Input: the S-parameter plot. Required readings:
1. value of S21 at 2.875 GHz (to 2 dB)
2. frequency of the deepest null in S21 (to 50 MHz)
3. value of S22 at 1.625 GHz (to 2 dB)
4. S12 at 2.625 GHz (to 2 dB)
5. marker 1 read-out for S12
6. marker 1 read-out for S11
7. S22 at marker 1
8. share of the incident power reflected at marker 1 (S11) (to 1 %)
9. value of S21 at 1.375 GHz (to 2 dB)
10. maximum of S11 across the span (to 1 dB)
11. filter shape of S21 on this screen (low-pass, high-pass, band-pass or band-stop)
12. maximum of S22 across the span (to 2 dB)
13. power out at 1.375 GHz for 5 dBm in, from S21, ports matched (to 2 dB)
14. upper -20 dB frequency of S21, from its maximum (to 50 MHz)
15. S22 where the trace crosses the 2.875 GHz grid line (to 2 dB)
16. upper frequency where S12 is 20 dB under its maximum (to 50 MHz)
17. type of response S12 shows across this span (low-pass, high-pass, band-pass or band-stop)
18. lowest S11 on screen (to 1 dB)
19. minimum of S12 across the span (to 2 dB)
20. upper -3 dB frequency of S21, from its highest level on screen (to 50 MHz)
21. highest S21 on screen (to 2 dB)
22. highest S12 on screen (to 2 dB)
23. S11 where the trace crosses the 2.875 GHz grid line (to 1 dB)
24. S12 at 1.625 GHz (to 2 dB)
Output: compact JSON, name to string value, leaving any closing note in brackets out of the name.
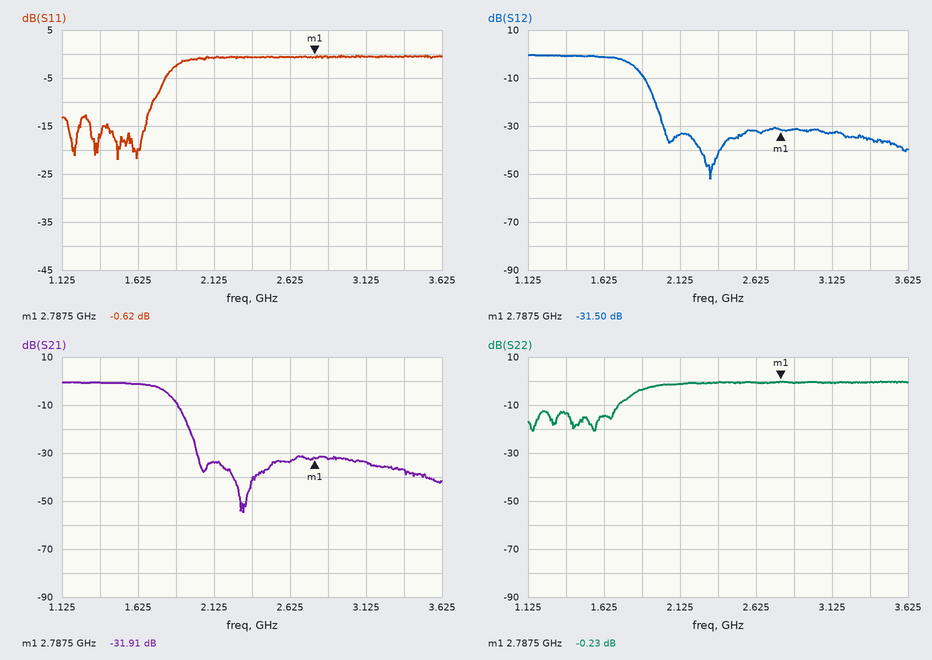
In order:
{"value of S21 at 2.875 GHz": "-32 dB", "frequency of the deepest null in S21": "2.30 GHz", "value of S22 at 1.625 GHz": "-14 dB", "S12 at 2.625 GHz": "-32 dB", "marker 1 read-out for S12": "-31.50 dB", "marker 1 read-out for S11": "-0.62 dB", "S22 at marker 1": "-0.23 dB", "share of the incident power reflected at marker 1 (S11)": "87 %", "value of S21 at 1.375 GHz": "0 dB", "maximum of S11 across the span": "0 dB", "filter shape of S21 on this screen": "low-pass", "maximum of S22 across the span": "0 dB", "power out at 1.375 GHz for 5 dBm in, from S21, ports matched": "4 dBm", "upper -20 dB frequency of S21, from its maximum": "1.95 GHz", "S22 where the trace crosses the 2.875 GHz grid line": "0 dB", "upper frequency where S12 is 20 dB under its maximum": "1.95 GHz", "type of response S12 shows across this span": "low-pass", "lowest S11 on screen": "-22 dB", "minimum of S12 across the span": "-52 dB", "upper -3 dB frequency of S21, from its highest level on screen": "1.80 GHz", "highest S21 on screen": "0 dB", "highest S12 on screen": "0 dB", "S11 where the trace crosses the 2.875 GHz grid line": "-1 dB", "S12 at 1.625 GHz": "-2 dB"}
